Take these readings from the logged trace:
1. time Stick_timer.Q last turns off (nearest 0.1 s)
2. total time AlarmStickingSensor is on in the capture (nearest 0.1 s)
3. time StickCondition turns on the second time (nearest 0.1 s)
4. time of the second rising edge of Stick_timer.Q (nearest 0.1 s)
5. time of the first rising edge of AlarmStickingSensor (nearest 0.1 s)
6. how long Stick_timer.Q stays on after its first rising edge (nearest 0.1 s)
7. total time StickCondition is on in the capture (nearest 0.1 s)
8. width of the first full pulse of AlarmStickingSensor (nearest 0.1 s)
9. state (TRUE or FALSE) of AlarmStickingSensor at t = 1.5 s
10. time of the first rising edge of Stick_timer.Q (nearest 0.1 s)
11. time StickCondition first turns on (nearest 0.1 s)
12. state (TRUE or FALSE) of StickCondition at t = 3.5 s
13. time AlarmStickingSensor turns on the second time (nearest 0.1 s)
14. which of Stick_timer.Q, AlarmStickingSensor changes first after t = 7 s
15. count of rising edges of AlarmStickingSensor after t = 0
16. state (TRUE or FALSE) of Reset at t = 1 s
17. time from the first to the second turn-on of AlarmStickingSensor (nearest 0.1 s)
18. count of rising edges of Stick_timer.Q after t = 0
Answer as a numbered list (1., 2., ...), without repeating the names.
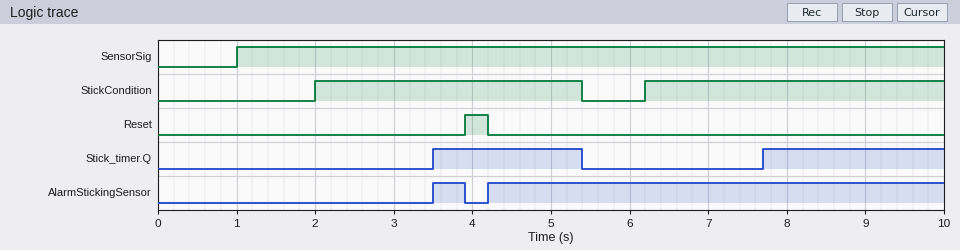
1. 5.4 s
2. 6.2 s
3. 6.2 s
4. 7.7 s
5. 3.5 s
6. 1.9 s
7. 7.2 s
8. 0.4 s
9. FALSE
10. 3.5 s
11. 2.0 s
12. TRUE
13. 4.2 s
14. Stick_timer.Q
15. 2
16. FALSE
17. 0.7 s
18. 2
